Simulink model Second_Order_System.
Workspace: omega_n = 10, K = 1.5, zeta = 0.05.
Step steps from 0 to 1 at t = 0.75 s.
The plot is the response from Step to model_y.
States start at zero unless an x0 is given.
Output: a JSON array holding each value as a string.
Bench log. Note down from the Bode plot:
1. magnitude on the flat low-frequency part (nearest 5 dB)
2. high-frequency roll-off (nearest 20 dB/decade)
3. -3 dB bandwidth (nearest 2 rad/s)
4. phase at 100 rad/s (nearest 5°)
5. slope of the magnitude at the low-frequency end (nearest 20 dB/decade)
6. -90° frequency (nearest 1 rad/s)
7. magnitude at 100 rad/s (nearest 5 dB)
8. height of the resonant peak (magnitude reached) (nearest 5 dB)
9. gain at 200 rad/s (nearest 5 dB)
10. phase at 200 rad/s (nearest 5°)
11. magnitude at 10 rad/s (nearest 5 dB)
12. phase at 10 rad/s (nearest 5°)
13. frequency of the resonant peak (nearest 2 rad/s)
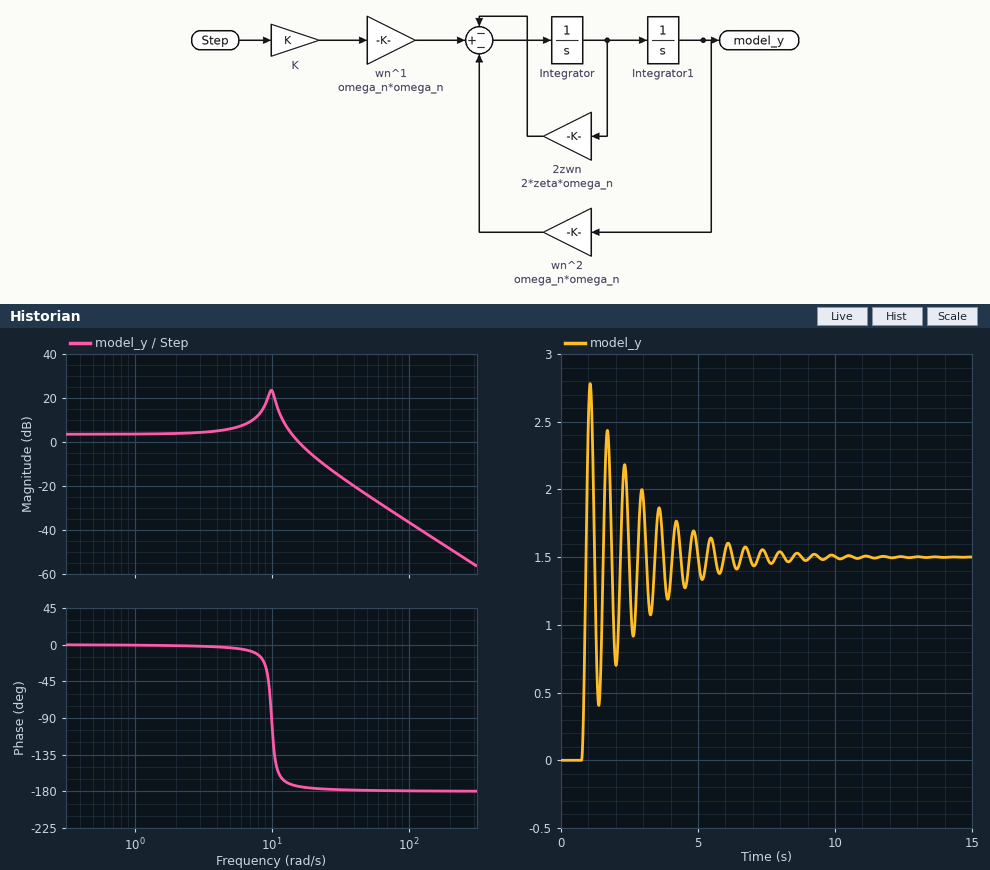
["5 dB", "-40 dB/decade", "16 rad/s", "-180°", "0 dB/decade", "10 rad/s", "-35 dB", "25 dB", "-50 dB", "-180°", "25 dB", "-90°", "10 rad/s"]
